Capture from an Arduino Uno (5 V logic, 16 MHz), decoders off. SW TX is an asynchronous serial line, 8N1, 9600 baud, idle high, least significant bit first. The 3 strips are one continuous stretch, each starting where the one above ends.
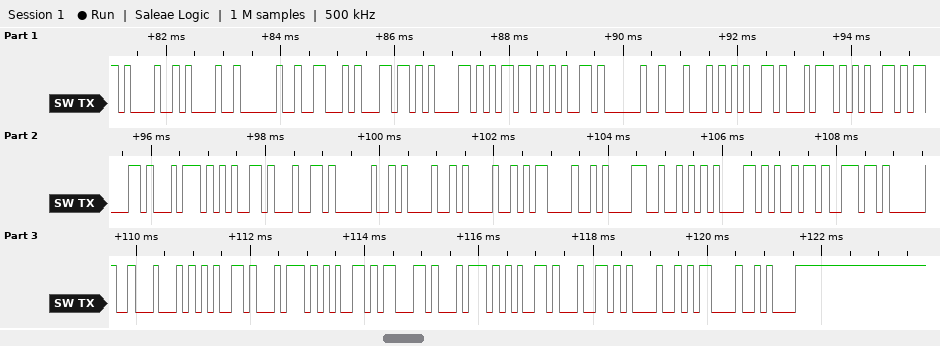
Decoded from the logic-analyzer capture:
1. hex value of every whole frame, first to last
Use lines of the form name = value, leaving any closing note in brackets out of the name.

hex value of every whole frame, first to last = 21 21 20 46 6C 61 6D 65 20 44 65 74 65 63 74 65 64 20 21 21 0D 0A 52 61 69 6E 20 44 65 74 65 63 74 65 64 21 0D 0A
